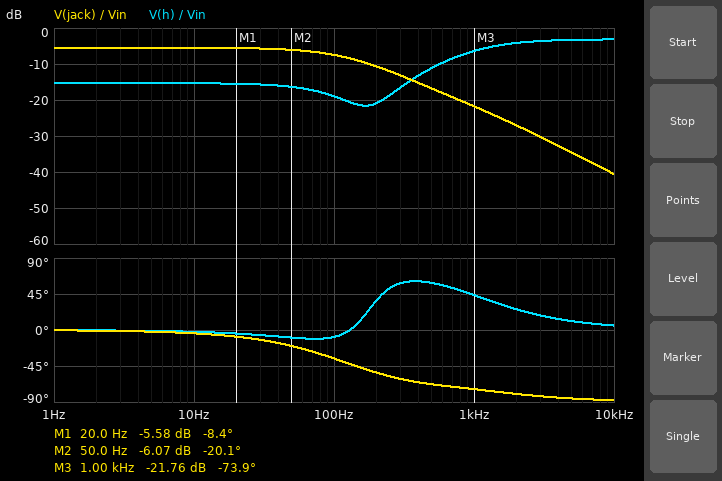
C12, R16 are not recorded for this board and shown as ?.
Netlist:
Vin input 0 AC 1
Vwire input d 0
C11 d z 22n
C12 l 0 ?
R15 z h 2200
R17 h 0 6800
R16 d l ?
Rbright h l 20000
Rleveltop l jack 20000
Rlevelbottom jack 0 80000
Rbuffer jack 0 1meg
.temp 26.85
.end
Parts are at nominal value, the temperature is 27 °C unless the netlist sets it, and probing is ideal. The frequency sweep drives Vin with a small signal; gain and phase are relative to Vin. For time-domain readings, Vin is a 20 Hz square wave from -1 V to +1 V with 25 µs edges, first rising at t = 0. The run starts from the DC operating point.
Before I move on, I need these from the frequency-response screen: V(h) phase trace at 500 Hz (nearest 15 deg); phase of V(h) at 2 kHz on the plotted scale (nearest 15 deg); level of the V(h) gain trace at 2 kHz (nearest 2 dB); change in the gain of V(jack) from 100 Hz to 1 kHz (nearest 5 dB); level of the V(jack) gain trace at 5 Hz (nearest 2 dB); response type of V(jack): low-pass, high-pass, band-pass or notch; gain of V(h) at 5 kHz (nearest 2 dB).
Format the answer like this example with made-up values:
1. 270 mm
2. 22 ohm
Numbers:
1. 60 deg
2. 30 deg
3. -4 dB
4. -15 dB
5. -6 dB
6. low-pass
7. -4 dB
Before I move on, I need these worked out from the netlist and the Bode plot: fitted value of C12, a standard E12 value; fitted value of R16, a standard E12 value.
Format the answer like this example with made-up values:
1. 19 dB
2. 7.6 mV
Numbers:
1. 180 nF
2. 10 kΩ
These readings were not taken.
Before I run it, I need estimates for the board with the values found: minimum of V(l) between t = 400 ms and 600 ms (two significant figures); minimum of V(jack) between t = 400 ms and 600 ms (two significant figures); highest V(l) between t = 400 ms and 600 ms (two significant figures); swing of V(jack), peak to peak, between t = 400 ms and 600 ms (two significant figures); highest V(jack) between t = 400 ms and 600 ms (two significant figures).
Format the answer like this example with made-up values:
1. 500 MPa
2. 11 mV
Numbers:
1. -680 mV
2. -530 mV
3. 680 mV
4. 1.1 V
5. 530 mV
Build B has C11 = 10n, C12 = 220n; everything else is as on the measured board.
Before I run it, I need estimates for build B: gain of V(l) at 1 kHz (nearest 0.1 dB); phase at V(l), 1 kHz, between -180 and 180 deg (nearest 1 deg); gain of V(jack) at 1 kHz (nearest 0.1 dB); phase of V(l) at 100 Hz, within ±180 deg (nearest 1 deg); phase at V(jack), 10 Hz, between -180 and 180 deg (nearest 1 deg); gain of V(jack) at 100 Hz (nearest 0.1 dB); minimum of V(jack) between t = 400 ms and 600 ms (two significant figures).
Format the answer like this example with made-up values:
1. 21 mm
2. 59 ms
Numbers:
1. -22.3 dB
2. -77 deg
3. -24.4 dB
4. -42 deg
5. -5 deg
6. -8.2 dB
7. -530 mV
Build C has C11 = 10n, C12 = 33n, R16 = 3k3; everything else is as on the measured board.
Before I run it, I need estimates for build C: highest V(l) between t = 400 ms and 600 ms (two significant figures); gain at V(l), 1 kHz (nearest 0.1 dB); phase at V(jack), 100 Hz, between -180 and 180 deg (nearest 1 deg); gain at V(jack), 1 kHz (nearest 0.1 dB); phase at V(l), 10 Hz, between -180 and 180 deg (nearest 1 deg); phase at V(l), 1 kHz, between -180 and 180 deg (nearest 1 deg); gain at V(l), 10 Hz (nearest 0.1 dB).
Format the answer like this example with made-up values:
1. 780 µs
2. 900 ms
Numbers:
1. 860 mV
2. -2.5 dB
3. -3 deg
4. -4.5 dB
5. 0 deg
6. -28 deg
7. -1.3 dB
